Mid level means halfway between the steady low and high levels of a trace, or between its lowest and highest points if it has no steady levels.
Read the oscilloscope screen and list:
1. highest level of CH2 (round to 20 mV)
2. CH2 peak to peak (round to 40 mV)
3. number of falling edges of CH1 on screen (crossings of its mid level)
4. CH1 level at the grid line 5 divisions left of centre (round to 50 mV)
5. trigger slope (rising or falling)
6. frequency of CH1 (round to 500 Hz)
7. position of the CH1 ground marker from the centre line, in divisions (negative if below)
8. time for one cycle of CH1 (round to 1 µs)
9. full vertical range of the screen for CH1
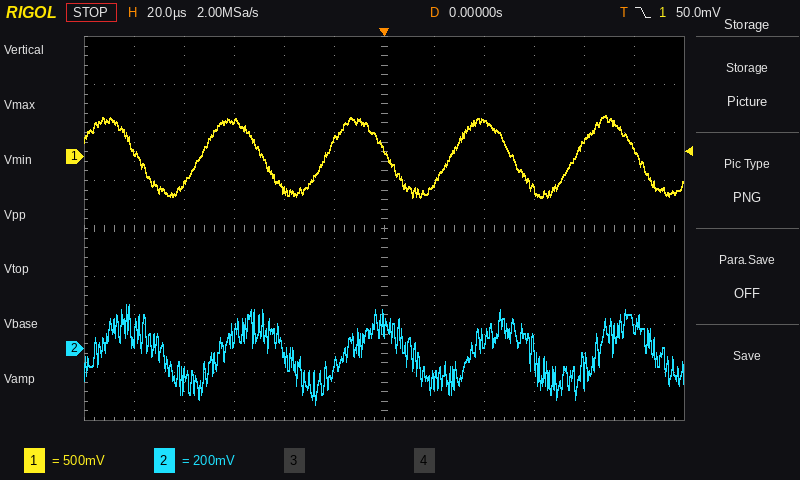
180 mV
400 mV
5
50 mV
falling
20.0 kHz
+1.5 div
50 µs
4 V
